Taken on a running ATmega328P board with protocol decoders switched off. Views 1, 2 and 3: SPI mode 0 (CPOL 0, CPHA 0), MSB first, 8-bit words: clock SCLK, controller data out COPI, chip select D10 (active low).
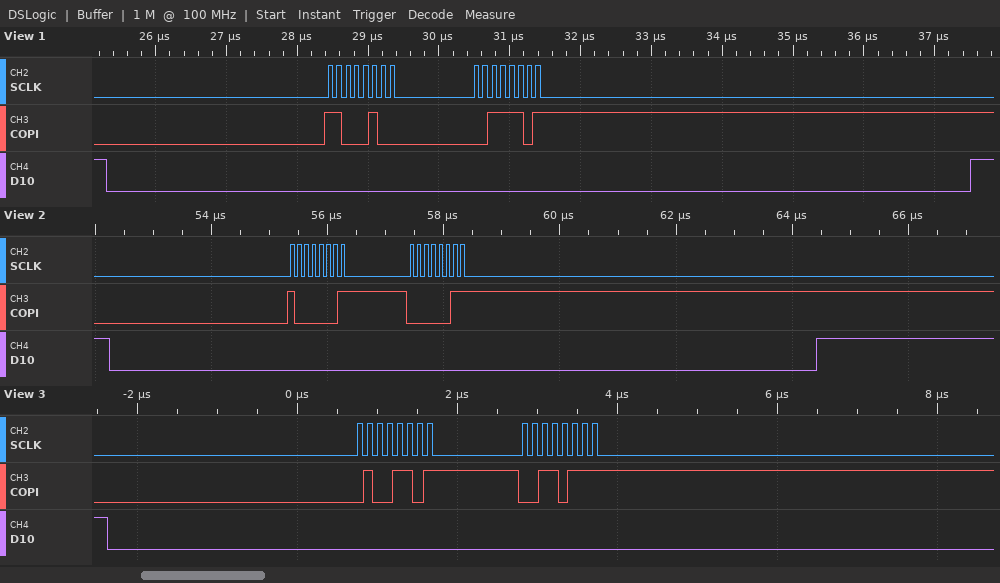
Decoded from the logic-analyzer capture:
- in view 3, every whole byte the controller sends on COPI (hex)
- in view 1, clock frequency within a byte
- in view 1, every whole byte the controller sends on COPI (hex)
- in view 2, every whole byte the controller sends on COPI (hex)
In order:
4D 37
8 MHz
C4 3D
81 03
